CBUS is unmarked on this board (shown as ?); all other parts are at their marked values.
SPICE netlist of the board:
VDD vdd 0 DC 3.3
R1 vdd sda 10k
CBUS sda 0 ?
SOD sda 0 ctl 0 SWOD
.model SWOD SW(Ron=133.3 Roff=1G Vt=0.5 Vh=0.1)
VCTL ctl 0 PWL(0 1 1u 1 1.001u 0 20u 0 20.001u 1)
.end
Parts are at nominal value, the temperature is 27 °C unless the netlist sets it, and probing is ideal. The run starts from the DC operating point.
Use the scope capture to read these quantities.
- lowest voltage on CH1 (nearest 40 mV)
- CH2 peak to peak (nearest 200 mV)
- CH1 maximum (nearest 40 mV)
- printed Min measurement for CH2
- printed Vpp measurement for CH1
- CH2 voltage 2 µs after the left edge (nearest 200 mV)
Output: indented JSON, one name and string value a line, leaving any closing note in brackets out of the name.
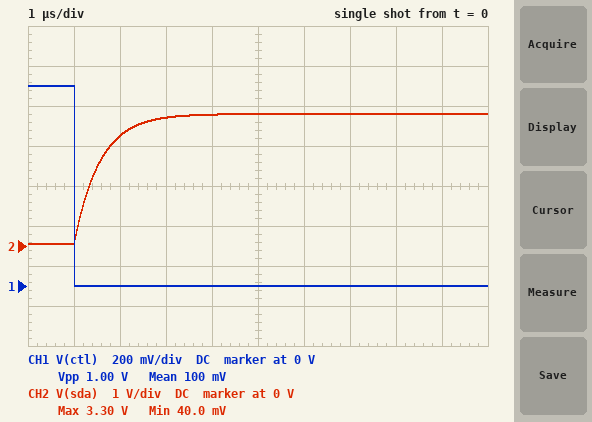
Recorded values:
{
  "lowest voltage on CH1": "0 V",
  "CH2 peak to peak": "3.2 V",
  "CH1 maximum": "1.00 V",
  "printed Min measurement for CH2": "40.0 mV",
  "printed Vpp measurement for CH1": "1.00 V",
  "CH2 voltage 2 µs after the left edge": "2.8 V"
}
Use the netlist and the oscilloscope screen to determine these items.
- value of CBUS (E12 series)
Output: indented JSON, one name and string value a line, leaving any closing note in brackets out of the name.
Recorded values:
{
  "value of CBUS": "56 pF"
}
